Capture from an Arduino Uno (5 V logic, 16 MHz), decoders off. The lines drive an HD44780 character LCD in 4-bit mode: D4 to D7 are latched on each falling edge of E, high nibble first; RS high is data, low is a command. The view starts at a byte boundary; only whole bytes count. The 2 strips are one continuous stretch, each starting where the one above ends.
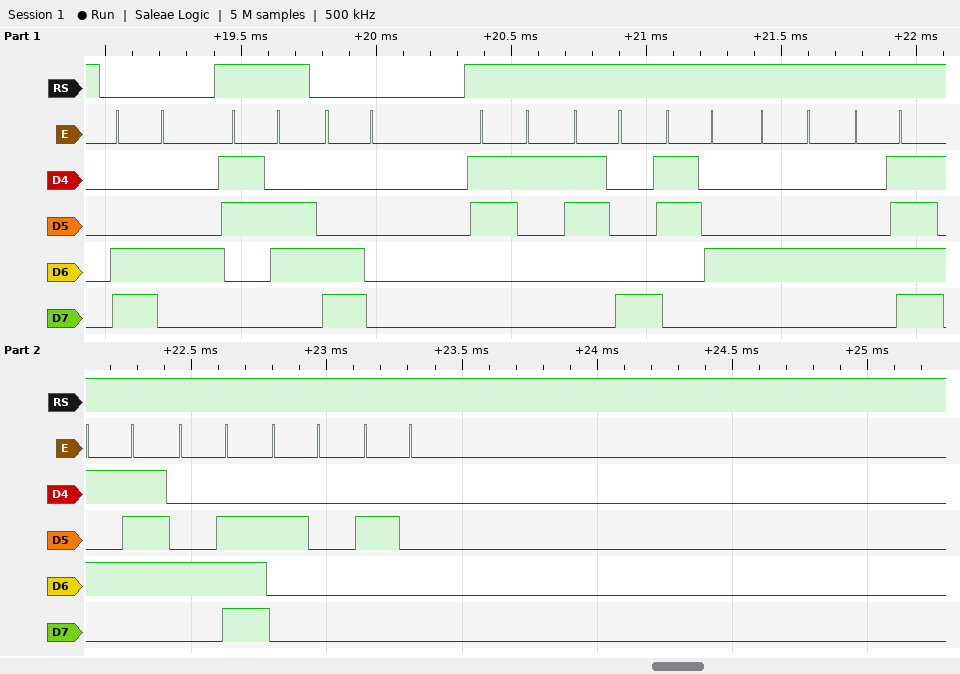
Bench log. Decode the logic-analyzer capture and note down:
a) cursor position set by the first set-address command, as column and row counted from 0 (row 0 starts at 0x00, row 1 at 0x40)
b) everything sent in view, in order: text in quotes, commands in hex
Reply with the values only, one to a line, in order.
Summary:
column 4, row 1
0xC4 "6" 0xC0 "184DOWN  "
